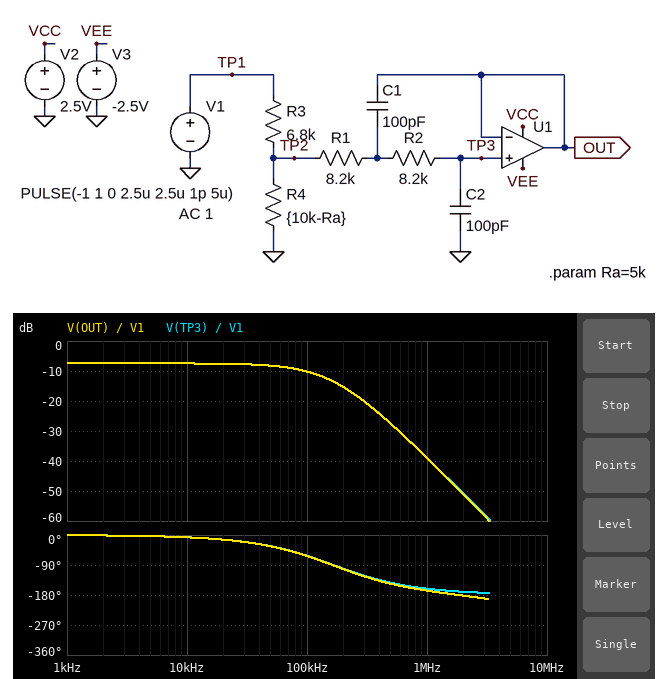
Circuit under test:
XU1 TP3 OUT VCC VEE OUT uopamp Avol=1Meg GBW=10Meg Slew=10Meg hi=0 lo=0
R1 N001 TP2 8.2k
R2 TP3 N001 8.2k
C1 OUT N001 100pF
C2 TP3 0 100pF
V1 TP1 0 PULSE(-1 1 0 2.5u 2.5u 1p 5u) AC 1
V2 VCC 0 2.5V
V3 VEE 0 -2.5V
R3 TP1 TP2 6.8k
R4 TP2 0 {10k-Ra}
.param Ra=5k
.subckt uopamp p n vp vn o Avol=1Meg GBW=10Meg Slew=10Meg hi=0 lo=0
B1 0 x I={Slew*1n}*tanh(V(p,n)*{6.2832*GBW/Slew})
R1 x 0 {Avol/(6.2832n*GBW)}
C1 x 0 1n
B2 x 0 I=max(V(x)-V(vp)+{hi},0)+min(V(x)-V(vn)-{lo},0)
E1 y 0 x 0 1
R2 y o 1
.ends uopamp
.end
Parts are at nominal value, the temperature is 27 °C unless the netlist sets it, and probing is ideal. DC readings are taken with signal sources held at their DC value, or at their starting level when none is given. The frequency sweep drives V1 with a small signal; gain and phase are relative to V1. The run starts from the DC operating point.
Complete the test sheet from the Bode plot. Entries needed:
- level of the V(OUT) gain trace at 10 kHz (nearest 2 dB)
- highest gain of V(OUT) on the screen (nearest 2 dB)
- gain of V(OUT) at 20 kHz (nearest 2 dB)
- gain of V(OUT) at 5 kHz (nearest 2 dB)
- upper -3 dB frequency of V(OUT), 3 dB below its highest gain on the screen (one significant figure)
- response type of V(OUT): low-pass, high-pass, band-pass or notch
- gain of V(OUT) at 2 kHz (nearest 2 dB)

-8 dB
-8 dB
-8 dB
-8 dB
100 kHz
low-pass
-8 dB
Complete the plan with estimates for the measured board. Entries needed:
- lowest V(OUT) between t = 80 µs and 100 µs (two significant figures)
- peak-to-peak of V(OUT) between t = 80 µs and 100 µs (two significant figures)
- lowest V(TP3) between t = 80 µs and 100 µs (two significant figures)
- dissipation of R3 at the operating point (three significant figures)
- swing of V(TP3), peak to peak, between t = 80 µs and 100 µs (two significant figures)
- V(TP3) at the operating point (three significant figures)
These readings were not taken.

-140 mV
270 mV
-140 mV
48.8 µW
270 mV
-424 mV
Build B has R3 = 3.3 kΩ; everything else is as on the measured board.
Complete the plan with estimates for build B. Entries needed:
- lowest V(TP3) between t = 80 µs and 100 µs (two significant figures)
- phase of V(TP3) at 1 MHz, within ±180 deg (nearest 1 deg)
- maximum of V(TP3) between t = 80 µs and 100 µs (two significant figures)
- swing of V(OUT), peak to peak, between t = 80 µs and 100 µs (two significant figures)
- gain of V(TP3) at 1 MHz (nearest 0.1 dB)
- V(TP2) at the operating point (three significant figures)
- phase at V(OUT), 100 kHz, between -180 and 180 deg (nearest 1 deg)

-210 mV
-160 deg
210 mV
410 mV
-35.2 dB
-602 mV
-61 deg
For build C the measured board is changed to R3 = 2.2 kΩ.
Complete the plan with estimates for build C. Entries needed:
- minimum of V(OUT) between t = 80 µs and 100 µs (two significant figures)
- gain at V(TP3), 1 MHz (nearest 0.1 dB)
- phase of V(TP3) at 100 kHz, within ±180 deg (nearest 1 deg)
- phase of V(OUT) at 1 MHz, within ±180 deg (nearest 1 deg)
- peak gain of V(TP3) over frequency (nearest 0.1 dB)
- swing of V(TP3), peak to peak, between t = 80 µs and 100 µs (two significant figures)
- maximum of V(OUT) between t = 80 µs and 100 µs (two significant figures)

-240 mV
-33.6 dB
-59 deg
-166 deg
-3.2 dB
490 mV
240 mV
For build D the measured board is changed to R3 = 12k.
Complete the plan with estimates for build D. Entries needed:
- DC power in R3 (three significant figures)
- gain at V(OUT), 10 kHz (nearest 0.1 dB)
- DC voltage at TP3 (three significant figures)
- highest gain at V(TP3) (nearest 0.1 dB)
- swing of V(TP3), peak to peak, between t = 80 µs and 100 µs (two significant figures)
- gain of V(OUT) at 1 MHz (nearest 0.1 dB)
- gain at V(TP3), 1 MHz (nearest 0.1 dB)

41.5 µW
-10.7 dB
-294 mV
-10.6 dB
180 mV
-42.7 dB
-42.6 dB
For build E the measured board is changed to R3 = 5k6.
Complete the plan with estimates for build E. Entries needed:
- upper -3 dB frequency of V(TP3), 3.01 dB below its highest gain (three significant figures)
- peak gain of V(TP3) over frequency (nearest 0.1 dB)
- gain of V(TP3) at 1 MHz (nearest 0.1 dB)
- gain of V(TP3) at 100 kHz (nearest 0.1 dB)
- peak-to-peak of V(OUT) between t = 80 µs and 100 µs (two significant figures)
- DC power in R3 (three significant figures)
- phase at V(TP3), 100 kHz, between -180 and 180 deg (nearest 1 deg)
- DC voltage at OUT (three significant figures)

108 kHz
-6.5 dB
-37.8 dB
-9.2 dB
310 mV
49.8 µW
-62 deg
-472 mV
